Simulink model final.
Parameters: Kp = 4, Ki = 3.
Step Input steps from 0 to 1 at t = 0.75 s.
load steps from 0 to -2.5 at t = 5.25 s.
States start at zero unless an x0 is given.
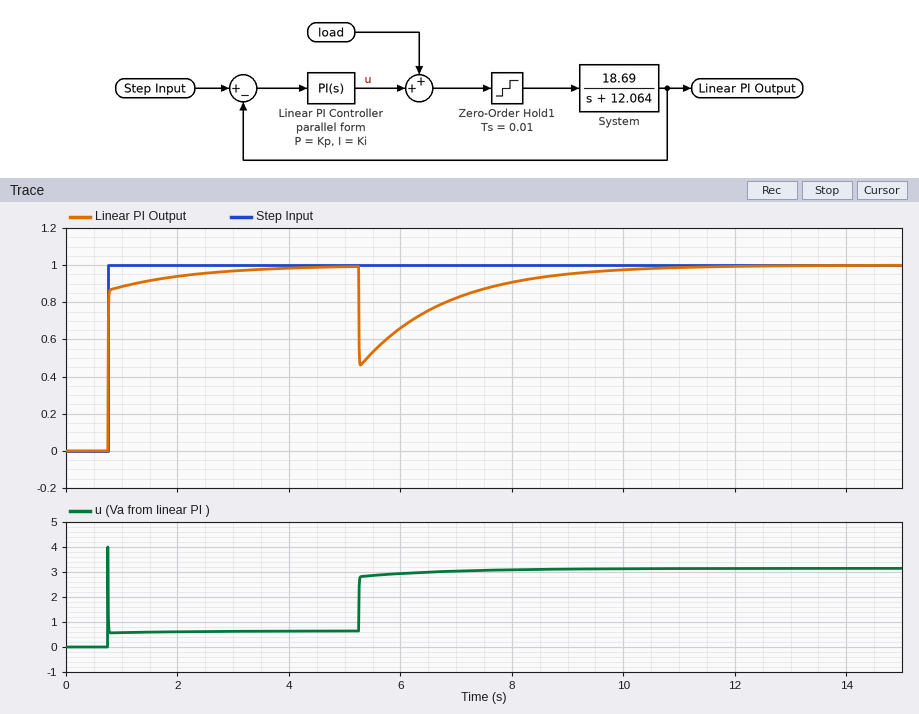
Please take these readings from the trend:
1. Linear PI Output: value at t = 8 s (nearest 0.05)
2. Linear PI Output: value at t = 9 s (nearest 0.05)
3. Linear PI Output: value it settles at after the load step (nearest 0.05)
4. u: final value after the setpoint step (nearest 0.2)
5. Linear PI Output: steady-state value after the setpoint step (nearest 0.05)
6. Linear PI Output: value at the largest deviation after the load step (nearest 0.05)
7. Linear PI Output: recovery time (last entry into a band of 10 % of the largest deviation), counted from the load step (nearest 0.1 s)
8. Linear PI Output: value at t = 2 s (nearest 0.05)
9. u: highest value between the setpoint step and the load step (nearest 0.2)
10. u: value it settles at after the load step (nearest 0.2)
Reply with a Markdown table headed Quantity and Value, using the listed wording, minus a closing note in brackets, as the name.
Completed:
| Quantity | Value |
|---|---|
| Linear PI Output: value at t = 8 s | 0.90 |
| Linear PI Output: value at t = 9 s | 0.95 |
| Linear PI Output: value it settles at after the load step | 1.00 |
| u: final value after the setpoint step | 0.6 |
| Linear PI Output: steady-state value after the setpoint step | 1.00 |
| Linear PI Output: value at the largest deviation after the load step | 0.45 |
| Linear PI Output: recovery time (last entry into a band of 10 % of the largest deviation), counted from the load step | 3.6 s |
| Linear PI Output: value at t = 2 s | 0.95 |
| u: highest value between the setpoint step and the load step | 4.0 |
| u: value it settles at after the load step | 3.2 |
